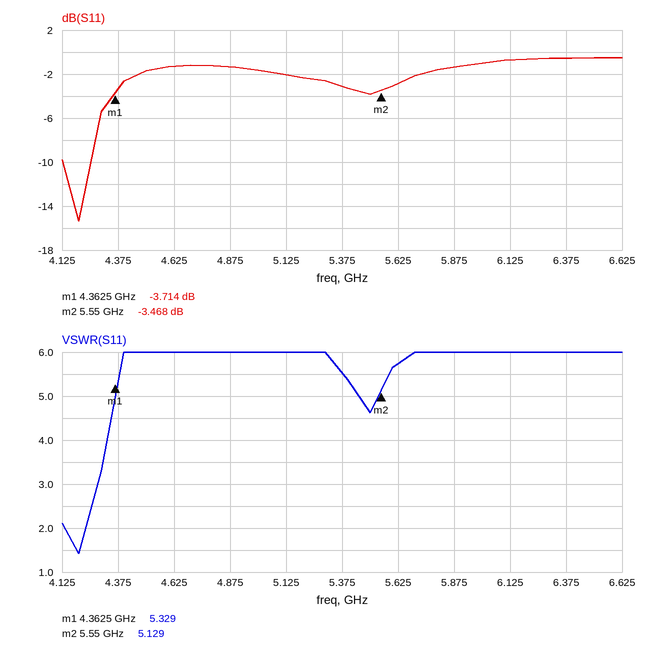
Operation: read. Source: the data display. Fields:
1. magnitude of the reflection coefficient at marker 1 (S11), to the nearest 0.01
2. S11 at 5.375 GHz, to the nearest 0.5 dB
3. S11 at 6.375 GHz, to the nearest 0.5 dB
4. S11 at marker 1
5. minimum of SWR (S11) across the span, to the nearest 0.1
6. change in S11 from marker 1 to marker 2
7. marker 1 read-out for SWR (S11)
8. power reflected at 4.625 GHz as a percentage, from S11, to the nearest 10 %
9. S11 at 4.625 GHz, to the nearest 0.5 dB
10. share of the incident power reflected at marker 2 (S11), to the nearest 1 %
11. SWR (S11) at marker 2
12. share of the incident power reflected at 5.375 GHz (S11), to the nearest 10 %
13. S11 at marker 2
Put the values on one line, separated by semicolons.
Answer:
0.65; -3.0 dB; -0.5 dB; -3.714 dB; 1.4; 0.246 dB; 5.329; 70 %; -1.5 dB; 45 %; 5.129; 50 %; -3.468 dB
